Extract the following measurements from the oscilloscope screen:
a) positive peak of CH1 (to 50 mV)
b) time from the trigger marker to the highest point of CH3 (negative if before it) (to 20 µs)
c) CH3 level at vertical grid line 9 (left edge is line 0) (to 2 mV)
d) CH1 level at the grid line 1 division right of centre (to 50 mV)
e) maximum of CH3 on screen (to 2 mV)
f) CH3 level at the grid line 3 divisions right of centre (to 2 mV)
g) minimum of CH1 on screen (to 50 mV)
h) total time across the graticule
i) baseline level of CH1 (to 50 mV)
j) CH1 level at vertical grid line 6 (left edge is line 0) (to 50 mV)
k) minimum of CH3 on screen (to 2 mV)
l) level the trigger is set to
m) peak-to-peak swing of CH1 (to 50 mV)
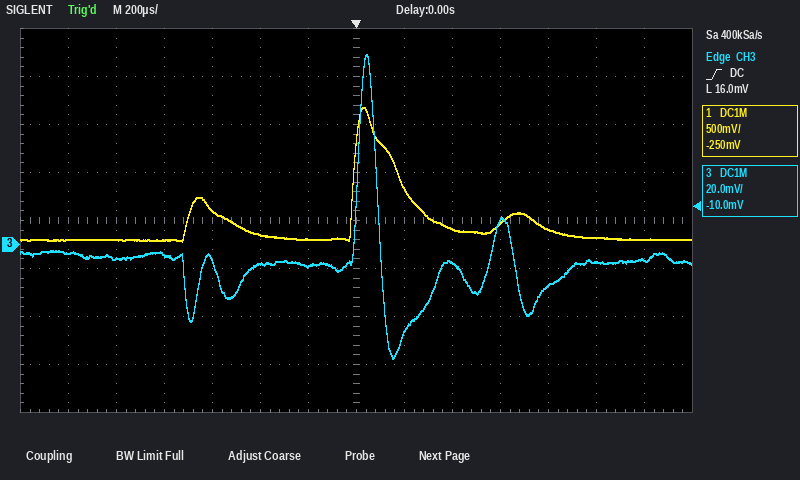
1.45 V
+40 µs
-8 mV
600 mV
80 mV
10 mV
50 mV
2.8 ms
50 mV
50 mV
-48 mV
16.0 mV
1.40 V
